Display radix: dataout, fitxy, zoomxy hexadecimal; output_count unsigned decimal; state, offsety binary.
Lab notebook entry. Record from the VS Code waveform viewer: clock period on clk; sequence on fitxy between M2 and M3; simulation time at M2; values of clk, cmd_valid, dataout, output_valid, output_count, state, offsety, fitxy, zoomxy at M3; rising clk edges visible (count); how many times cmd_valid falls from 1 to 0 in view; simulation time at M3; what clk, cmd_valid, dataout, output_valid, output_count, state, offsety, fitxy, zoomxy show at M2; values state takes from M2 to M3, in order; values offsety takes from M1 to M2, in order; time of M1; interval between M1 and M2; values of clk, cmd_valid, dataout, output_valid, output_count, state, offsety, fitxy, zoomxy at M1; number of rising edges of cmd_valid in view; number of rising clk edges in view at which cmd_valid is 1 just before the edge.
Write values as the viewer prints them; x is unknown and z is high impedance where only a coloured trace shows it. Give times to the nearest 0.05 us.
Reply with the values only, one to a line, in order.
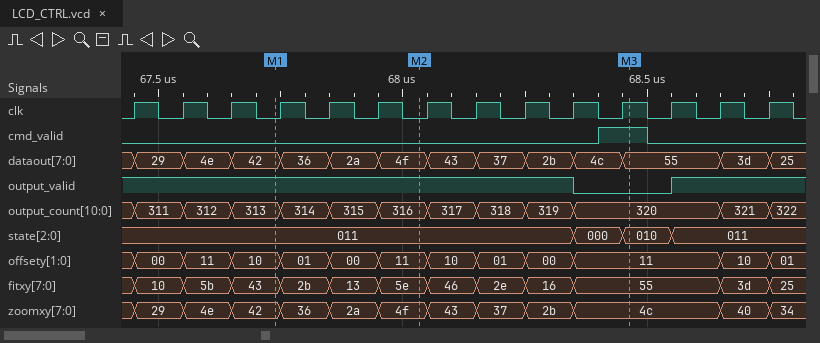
0.1 us
5e, 46, 2e, 16, 55
68.05 us
clk=1, cmd_valid=1, dataout=55, output_valid=0, output_count=320, state=010, offsety=11, fitxy=55, zoomxy=4c
14
1
68.45 us
clk=0, cmd_valid=0, dataout=4f, output_valid=1, output_count=316, state=011, offsety=11, fitxy=5e, zoomxy=4f
011, 000, 010
10, 01, 00, 11
67.75 us
0.3 us
clk=0, cmd_valid=0, dataout=42, output_valid=1, output_count=313, state=011, offsety=10, fitxy=43, zoomxy=42
1
1
